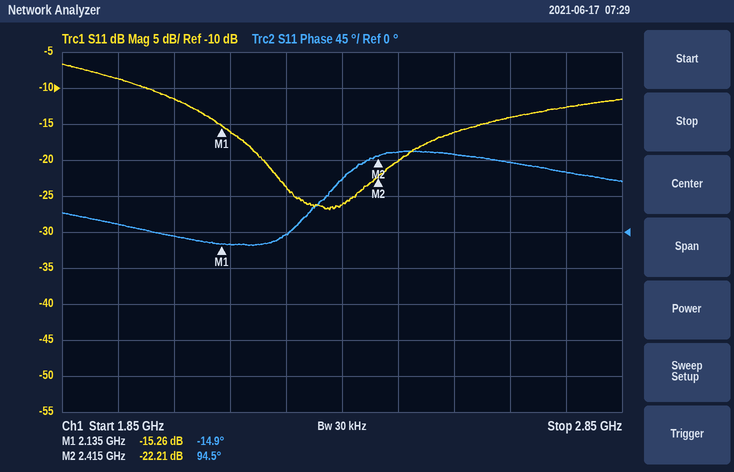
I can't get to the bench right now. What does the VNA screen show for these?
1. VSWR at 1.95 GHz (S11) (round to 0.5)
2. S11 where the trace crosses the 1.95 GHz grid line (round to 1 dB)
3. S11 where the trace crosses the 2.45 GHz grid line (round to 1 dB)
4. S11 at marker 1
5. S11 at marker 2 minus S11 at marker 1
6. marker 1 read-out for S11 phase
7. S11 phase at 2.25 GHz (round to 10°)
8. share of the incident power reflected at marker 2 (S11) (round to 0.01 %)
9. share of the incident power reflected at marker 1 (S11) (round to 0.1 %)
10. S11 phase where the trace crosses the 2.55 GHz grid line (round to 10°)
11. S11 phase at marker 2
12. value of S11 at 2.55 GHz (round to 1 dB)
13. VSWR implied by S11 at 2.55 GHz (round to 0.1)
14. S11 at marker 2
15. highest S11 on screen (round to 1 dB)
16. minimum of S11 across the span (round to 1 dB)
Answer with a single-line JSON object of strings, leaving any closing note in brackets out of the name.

{"VSWR at 1.95 GHz (S11)": "2.0", "S11 where the trace crosses the 1.95 GHz grid line": "-9 dB", "S11 where the trace crosses the 2.45 GHz grid line": "-20 dB", "S11 at marker 1": "-15.26 dB", "S11 at marker 2 minus S11 at marker 1": "-6.95 dB", "marker 1 read-out for S11 phase": "-14.9°", "S11 phase at 2.25 GHz": "0°", "share of the incident power reflected at marker 2 (S11)": "0.60 %", "share of the incident power reflected at marker 1 (S11)": "3.0 %", "S11 phase where the trace crosses the 2.55 GHz grid line": "100°", "S11 phase at marker 2": "94.5°", "value of S11 at 2.55 GHz": "-16 dB", "VSWR implied by S11 at 2.55 GHz": "1.4", "S11 at marker 2": "-22.21 dB", "highest S11 on screen": "-7 dB", "minimum of S11 across the span": "-27 dB"}
